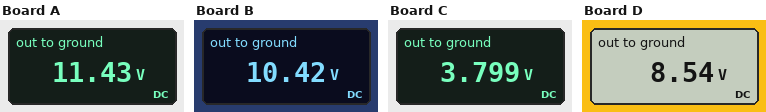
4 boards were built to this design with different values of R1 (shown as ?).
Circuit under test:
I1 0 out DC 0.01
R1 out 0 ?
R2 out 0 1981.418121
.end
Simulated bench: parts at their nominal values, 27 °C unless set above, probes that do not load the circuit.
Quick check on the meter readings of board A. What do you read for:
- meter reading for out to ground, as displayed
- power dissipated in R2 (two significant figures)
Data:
11.43 V
66 mW
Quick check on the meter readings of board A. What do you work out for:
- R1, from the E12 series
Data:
2.7 kΩ
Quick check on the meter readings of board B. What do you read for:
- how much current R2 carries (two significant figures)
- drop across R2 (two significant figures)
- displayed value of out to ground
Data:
5.3 mA
10 V
10.42 V
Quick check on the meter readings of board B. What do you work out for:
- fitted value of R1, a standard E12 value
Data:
2.2 kΩ
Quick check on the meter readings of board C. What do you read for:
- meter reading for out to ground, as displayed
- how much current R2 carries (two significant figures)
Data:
3.799 V
1.9 mA
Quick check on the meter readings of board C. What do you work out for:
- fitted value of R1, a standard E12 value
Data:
470 Ω
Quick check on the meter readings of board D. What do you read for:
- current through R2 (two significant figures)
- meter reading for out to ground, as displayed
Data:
4.3 mA
8.54 V
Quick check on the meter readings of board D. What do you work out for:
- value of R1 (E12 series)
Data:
1.5 kΩ
